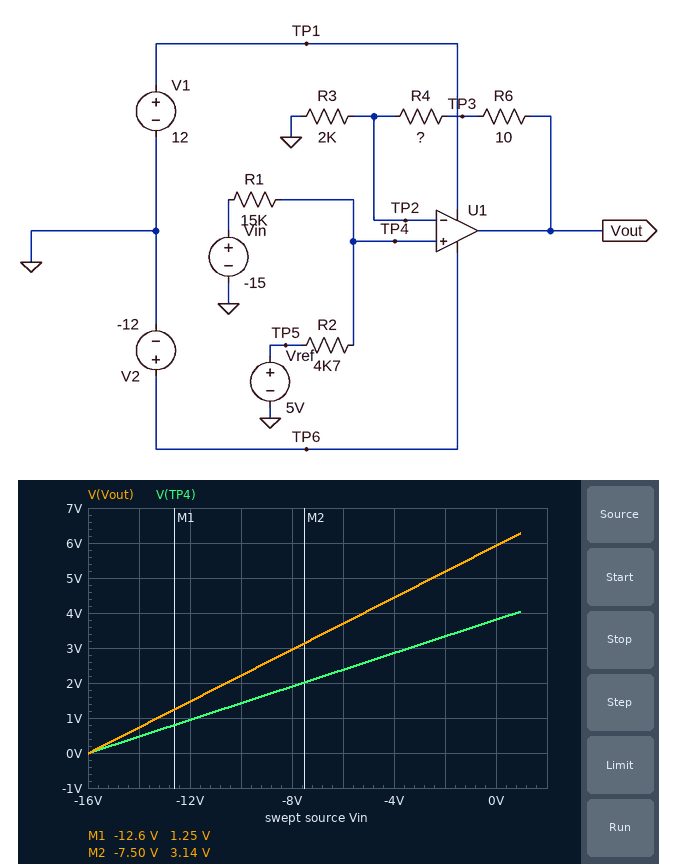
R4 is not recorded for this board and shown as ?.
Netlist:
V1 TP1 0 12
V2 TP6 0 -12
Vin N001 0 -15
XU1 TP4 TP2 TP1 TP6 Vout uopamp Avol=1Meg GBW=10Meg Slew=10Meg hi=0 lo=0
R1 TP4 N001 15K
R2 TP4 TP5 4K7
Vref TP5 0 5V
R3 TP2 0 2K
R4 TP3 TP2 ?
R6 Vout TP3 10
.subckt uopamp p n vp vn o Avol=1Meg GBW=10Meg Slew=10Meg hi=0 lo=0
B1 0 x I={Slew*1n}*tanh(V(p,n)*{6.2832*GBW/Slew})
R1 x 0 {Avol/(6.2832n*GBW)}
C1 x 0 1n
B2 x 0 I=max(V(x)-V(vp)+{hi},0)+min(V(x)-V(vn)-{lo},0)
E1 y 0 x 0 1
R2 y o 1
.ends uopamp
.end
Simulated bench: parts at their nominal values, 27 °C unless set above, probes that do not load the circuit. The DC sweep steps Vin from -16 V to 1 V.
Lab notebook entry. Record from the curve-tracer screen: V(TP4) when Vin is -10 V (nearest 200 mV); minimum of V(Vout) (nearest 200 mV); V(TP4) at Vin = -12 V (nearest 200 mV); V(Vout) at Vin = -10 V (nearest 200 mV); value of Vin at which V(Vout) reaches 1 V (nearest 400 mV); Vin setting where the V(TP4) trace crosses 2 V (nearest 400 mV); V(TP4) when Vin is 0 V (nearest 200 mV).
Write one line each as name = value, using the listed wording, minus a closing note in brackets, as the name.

V(TP4) when Vin is -10 V = 1.4 V
minimum of V(Vout) = 0 V
V(TP4) at Vin = -12 V = 1.0 V
V(Vout) at Vin = -10 V = 2.2 V
value of Vin at which V(Vout) reaches 1 V = -13.2 V
Vin setting where the V(TP4) trace crosses 2 V = -7.6 V
V(TP4) when Vin is 0 V = 3.8 V
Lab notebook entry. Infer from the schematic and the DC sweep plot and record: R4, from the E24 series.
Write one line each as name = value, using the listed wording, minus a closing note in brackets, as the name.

R4, from the E24 series = 1.1 kΩ
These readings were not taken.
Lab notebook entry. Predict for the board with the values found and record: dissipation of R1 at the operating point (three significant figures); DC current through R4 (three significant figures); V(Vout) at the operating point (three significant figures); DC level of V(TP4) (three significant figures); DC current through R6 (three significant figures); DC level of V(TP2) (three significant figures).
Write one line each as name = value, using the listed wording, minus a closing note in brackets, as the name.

dissipation of R1 at the operating point = 15.5 mW
DC current through R4 = 114 µA
V(Vout) at the operating point = 355 mV
DC level of V(TP4) = 228 mV
DC current through R6 = 114 µA
DC level of V(TP2) = 228 mV
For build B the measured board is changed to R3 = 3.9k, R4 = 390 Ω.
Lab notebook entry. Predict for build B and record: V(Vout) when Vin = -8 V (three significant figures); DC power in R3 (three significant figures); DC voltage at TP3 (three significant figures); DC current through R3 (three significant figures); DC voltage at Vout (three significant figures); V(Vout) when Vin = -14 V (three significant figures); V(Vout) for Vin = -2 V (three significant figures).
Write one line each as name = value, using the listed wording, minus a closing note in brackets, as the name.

V(Vout) when Vin = -8 V = 2.09 V
DC power in R3 = 13.4 µW
DC voltage at TP3 = 251 mV
DC current through R3 = 58.6 µA
DC voltage at Vout = 252 mV
V(Vout) when Vin = -14 V = 515 mV
V(Vout) for Vin = -2 V = 3.67 V
